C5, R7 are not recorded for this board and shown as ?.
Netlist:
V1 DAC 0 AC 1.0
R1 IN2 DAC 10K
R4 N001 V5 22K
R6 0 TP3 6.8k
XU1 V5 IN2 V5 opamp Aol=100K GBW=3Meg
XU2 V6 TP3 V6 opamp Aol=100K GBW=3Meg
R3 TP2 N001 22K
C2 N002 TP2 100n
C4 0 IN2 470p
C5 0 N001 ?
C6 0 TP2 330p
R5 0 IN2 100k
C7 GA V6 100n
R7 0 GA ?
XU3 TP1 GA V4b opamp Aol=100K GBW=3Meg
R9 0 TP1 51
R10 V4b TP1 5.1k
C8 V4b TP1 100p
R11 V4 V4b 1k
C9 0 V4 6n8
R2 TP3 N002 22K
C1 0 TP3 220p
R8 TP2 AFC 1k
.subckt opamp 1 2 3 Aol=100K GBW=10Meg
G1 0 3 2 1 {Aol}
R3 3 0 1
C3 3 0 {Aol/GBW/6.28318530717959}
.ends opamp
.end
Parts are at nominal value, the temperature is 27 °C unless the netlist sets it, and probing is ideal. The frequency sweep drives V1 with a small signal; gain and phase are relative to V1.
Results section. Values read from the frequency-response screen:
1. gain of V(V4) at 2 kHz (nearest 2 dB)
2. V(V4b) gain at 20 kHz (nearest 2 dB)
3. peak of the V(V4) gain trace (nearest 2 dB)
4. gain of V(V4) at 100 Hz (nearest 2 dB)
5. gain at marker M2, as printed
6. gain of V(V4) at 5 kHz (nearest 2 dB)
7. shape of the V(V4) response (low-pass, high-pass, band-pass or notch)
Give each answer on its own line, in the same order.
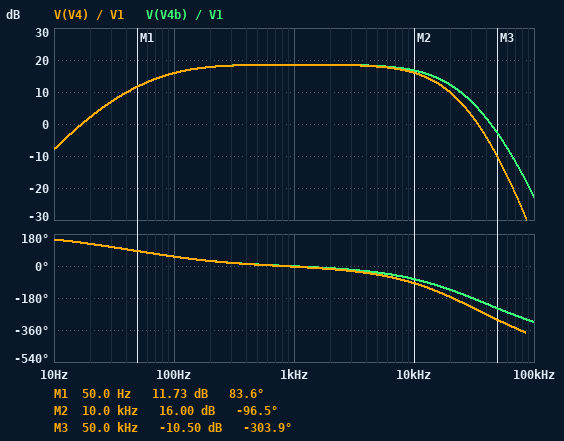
18 dB
12 dB
18 dB
16 dB
16.00 dB
18 dB
band-pass
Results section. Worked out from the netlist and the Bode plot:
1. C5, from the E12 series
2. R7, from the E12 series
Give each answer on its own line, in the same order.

270 pF
18 kΩ
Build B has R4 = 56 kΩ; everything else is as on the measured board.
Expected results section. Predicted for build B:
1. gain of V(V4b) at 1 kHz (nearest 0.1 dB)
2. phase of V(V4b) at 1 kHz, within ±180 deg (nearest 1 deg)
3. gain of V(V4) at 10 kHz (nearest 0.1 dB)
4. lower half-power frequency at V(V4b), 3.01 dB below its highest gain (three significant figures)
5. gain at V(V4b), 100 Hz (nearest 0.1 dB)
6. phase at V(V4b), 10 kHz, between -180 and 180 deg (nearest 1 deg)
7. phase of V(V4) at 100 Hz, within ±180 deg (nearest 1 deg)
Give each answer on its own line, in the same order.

15.2 dB
-3 deg
11.7 dB
89.4 Hz
12.7 dB
-85 deg
49 deg
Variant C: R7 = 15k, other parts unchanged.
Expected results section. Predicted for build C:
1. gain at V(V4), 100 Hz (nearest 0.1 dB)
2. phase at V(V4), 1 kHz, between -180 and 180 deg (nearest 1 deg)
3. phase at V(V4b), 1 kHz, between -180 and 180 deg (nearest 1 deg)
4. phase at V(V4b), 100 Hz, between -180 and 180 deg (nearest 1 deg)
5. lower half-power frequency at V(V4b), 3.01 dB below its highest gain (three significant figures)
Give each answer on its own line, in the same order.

15.2 dB
-3 deg
0 deg
58 deg
109 Hz
